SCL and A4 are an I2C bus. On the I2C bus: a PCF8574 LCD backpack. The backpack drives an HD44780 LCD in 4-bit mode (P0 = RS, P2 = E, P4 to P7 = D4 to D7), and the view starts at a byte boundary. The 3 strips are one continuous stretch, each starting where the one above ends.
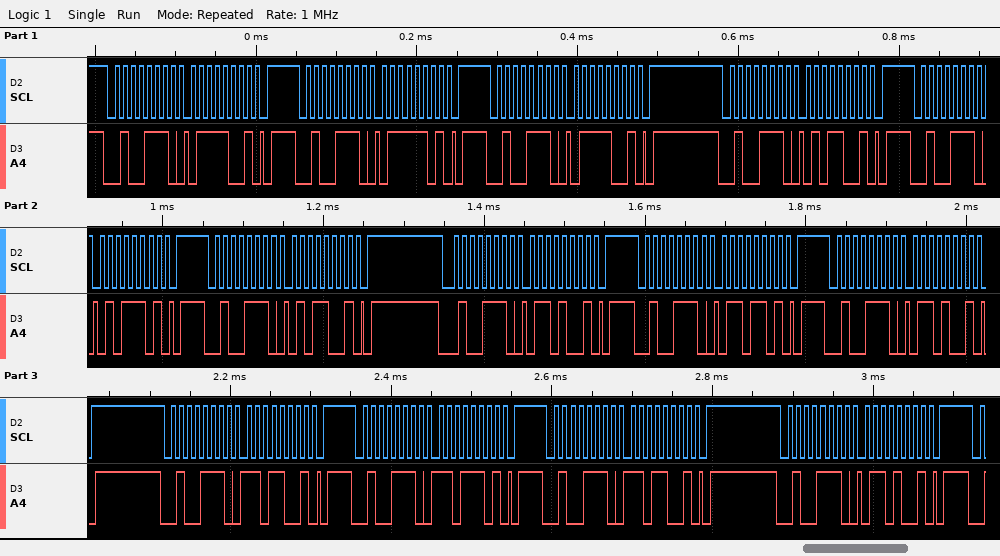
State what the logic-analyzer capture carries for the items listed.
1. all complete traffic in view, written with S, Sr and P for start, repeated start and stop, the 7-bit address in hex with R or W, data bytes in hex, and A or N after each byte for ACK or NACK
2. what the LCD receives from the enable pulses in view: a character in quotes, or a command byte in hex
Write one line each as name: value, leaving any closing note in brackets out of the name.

all complete traffic in view, written with S, Sr and P for start, repeated start and stop, the 7-bit address in hex with R or W, data bytes in hex, and A or N after each byte for ACK or NACK: S 27W A 79 A P S 27W A 7D A P S 27W A 79 A P S 27W A 59 A P S 27W A 5D A P S 27W A 59 A P S 27W A 69 A P S 27W A 6D A P S 27W A 69 A P S 27W A D9 A P S 27W A DD A P S 27W A D9 A P S 27W A 69 A P
what the LCD receives from the enable pulses in view: a character in quotes, or a command byte in hex: 'u' 'm'
